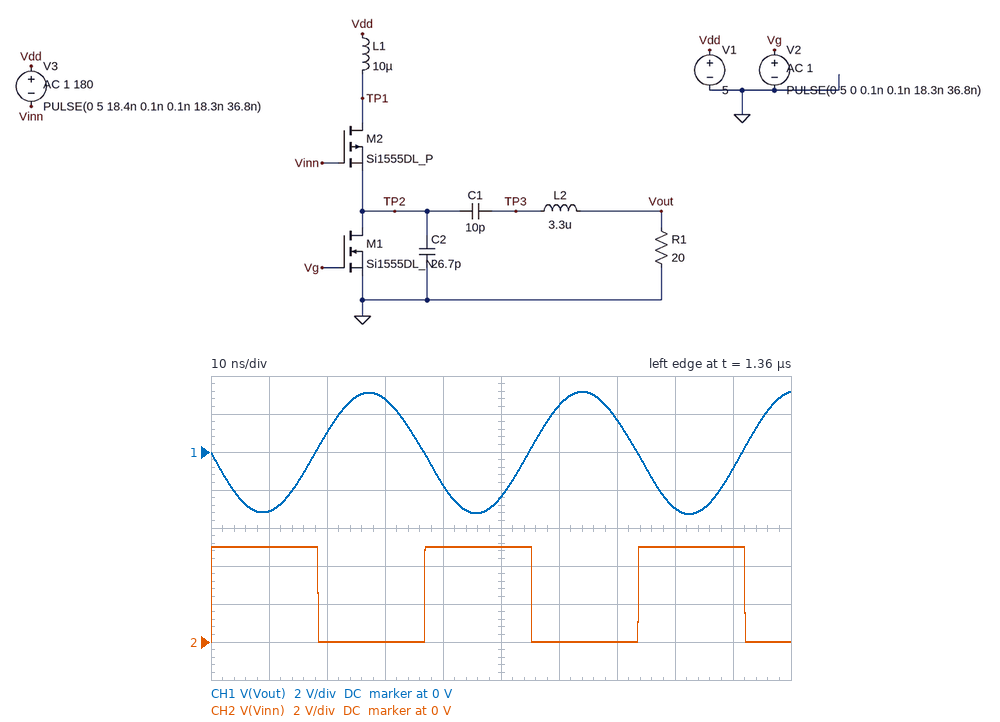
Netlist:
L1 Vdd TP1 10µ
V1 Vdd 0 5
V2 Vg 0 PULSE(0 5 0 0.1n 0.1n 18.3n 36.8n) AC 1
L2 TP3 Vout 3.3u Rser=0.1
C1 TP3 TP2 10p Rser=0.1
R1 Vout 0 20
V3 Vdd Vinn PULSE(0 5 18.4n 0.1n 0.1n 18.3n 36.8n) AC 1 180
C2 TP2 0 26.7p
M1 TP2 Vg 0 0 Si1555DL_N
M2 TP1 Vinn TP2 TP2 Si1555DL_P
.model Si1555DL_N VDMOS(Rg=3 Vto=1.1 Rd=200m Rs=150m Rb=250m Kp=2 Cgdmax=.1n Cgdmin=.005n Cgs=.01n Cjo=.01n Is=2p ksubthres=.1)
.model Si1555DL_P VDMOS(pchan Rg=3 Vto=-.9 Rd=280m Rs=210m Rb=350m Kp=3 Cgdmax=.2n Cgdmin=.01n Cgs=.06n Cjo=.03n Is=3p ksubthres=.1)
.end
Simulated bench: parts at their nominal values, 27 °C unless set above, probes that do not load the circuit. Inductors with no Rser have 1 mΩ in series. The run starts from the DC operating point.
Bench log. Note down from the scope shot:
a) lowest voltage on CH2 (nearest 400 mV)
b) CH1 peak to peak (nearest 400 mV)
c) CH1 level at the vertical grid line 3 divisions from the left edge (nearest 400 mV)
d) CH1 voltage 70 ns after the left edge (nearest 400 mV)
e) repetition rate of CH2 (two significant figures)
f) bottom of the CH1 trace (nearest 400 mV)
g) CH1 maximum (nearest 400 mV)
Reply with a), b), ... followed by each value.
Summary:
a) 0 V
b) 6.4 V
c) 2.8 V
d) 1.6 V
e) 27 MHz
f) -3.2 V
g) 3.2 V
